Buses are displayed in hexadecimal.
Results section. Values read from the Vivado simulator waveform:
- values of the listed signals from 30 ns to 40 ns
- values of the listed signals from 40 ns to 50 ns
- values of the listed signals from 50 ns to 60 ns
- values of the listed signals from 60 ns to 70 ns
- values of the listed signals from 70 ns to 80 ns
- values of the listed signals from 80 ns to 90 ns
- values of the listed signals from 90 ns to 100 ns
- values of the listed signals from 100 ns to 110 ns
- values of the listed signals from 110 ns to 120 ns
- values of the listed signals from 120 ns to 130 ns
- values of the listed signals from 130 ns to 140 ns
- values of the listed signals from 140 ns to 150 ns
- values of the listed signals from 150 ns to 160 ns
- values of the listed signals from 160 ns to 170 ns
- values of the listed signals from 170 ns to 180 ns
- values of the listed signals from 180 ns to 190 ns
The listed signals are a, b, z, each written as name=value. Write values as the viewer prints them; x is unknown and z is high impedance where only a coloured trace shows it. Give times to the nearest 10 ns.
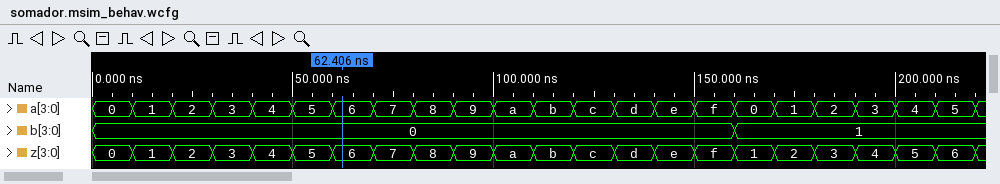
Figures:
a=3, b=0, z=3
a=4, b=0, z=4
a=5, b=0, z=5
a=6, b=0, z=6
a=7, b=0, z=7
a=8, b=0, z=8
a=9, b=0, z=9
a=a, b=0, z=a
a=b, b=0, z=b
a=c, b=0, z=c
a=d, b=0, z=d
a=e, b=0, z=e
a=f, b=0, z=f
a=0, b=1, z=1
a=1, b=1, z=2
a=2, b=1, z=3
